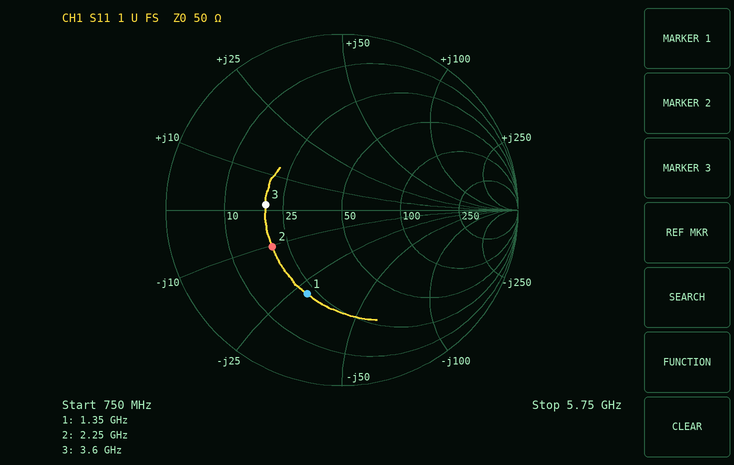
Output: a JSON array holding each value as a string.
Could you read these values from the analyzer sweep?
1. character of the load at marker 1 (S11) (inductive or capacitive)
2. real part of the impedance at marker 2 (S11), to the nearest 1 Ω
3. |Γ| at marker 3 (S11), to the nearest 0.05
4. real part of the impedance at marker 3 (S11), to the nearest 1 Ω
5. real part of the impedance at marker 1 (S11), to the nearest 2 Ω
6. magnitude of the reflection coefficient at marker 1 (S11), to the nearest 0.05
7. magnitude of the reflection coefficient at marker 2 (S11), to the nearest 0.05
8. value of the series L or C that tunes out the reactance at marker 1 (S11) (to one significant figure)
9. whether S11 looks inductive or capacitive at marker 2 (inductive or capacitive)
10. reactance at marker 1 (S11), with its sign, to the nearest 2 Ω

["capacitive", "20 Ω", "0.45", "20 Ω", "22 Ω", "0.50", "0.45", "3 nH", "capacitive", "-28 Ω"]
